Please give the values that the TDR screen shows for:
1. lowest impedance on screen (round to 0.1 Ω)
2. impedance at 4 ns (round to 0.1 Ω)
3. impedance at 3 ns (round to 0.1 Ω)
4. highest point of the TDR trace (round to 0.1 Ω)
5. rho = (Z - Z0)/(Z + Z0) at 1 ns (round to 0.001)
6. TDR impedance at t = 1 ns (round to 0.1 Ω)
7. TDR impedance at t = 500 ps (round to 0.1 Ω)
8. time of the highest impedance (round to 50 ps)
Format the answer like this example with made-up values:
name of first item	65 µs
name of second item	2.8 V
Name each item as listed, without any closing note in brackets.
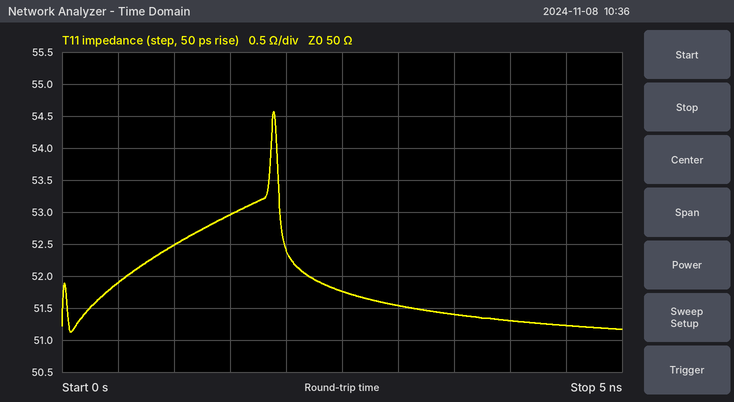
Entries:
lowest impedance on screen	51.1 Ω
impedance at 4 ns	51.3 Ω
impedance at 3 ns	51.5 Ω
highest point of the TDR trace	54.6 Ω
rho = (Z - Z0)/(Z + Z0) at 1 ns	+0.024
TDR impedance at t = 1 ns	52.5 Ω
TDR impedance at t = 500 ps	51.9 Ω
time of the highest impedance	1.90 ns
